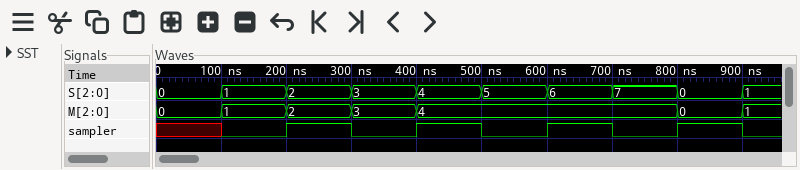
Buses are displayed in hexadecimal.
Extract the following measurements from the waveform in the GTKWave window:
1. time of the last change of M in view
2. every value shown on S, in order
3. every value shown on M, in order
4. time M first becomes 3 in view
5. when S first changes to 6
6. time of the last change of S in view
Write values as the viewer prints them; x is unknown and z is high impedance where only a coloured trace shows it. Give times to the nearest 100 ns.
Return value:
900 ns
0, 1, 2, 3, 4, 5, 6, 7, 0, 1
0, 1, 2, 3, 4, 0, 1
300 ns
600 ns
900 ns
